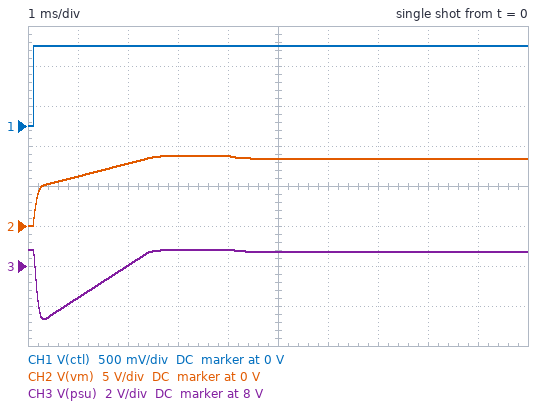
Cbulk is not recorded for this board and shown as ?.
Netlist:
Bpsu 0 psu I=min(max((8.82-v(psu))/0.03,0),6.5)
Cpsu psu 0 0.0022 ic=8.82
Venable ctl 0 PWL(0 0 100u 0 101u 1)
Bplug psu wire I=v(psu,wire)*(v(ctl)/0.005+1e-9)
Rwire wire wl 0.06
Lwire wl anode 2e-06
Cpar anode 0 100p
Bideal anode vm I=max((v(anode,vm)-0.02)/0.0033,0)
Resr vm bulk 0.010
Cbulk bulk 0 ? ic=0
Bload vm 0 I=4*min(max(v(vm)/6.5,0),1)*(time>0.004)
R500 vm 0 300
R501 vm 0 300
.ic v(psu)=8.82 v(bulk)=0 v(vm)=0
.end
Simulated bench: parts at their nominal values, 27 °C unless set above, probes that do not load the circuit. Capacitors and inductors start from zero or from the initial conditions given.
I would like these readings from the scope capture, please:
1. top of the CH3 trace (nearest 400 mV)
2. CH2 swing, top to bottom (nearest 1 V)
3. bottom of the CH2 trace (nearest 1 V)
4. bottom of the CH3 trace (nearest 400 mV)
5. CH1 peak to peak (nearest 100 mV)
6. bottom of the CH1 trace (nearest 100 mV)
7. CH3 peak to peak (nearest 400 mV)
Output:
8.8 V
9 V
0 V
5.2 V
1.0 V
0 V
3.6 V
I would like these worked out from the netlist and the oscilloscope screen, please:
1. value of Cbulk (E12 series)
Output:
1.8 mF
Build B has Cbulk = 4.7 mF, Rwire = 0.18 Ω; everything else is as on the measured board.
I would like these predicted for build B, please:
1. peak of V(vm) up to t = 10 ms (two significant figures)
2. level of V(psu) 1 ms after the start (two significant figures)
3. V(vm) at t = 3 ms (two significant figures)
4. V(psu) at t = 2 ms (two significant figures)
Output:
7.9 V
4.5 V
5.3 V
5.2 V
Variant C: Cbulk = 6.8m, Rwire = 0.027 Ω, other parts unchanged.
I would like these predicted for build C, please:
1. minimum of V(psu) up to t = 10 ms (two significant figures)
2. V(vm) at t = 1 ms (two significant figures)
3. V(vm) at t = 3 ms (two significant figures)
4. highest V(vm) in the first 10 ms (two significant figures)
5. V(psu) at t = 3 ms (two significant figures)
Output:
2.1 V
2.8 V
4.2 V
6.8 V
4.4 V
